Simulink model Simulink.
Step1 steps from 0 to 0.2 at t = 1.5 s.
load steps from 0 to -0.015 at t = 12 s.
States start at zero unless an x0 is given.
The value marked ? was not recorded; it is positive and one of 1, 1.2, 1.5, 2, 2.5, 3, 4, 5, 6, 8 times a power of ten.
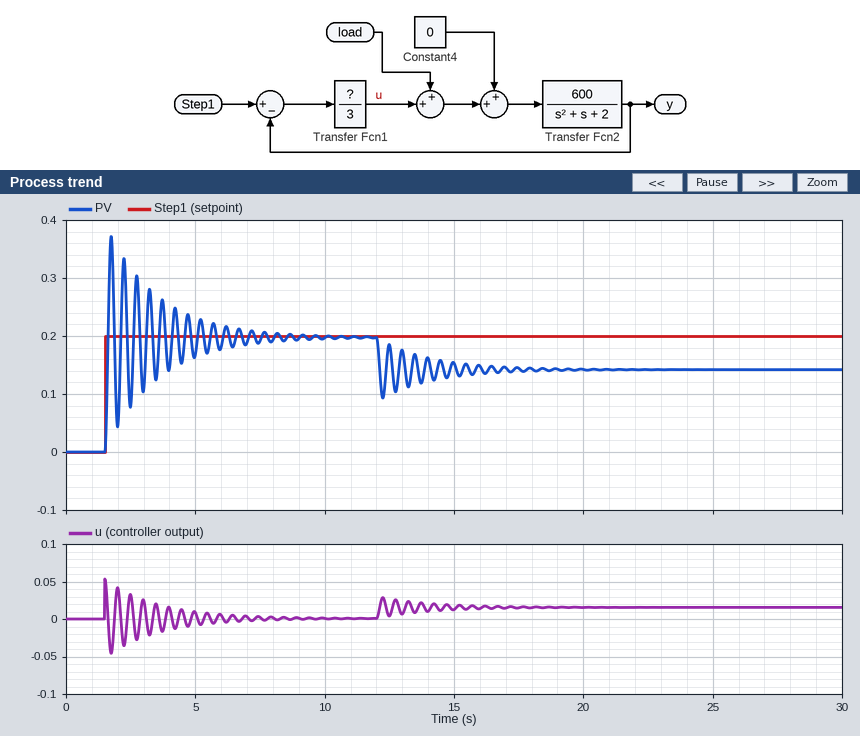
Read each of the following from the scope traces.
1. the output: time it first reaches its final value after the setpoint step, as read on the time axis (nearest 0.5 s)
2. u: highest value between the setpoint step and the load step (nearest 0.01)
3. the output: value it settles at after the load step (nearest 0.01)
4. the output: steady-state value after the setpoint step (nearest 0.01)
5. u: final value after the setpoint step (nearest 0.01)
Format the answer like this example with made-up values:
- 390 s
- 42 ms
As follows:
- 1.5 s
- 0.05
- 0.14
- 0.20
- 0.00
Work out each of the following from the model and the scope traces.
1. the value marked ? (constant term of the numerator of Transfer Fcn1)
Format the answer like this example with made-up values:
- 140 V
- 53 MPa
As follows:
- 0.8
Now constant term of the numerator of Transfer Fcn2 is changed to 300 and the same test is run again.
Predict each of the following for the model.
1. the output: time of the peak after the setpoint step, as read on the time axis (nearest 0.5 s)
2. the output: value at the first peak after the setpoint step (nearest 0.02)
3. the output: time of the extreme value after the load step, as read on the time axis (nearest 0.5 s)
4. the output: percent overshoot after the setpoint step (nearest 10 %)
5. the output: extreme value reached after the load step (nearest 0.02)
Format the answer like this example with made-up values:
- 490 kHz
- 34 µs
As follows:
- 2.0 s
- 0.36
- 12.5 s
- 80 %
- 0.10
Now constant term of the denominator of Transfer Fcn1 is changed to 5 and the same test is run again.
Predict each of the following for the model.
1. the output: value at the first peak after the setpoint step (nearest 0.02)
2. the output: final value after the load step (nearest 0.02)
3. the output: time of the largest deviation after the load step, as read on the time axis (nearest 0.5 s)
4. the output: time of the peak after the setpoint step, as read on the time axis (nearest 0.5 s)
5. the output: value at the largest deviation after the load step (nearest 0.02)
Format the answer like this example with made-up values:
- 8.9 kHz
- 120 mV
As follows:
- 0.36
- 0.10
- 12.5 s
- 2.0 s
- 0.02
